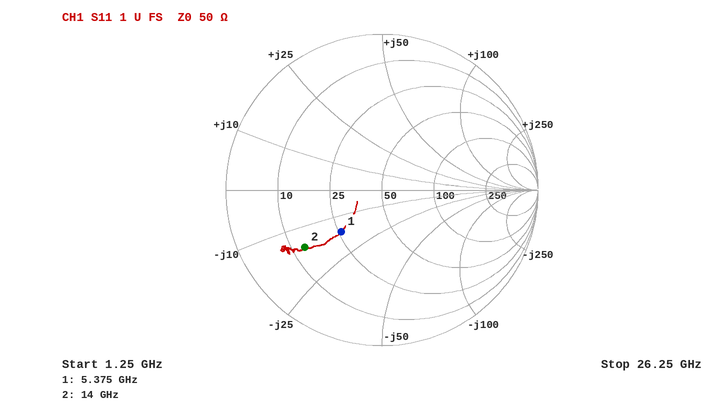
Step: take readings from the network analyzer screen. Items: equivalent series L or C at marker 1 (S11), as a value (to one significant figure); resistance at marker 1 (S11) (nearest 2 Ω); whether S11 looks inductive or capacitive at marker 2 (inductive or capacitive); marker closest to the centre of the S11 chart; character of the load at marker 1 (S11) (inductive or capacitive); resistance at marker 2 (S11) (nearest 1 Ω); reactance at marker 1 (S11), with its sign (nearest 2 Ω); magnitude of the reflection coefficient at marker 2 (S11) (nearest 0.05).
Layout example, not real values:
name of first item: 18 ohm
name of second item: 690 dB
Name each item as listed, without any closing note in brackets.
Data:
equivalent series L or C at marker 1 (S11), as a value: 2 pF
resistance at marker 1 (S11): 26 Ω
whether S11 looks inductive or capacitive at marker 2: capacitive
marker closest to the centre of the S11 chart: marker 1
character of the load at marker 1 (S11): capacitive
resistance at marker 2 (S11): 13 Ω
reactance at marker 1 (S11), with its sign: -16 Ω
magnitude of the reflection coefficient at marker 2 (S11): 0.60
